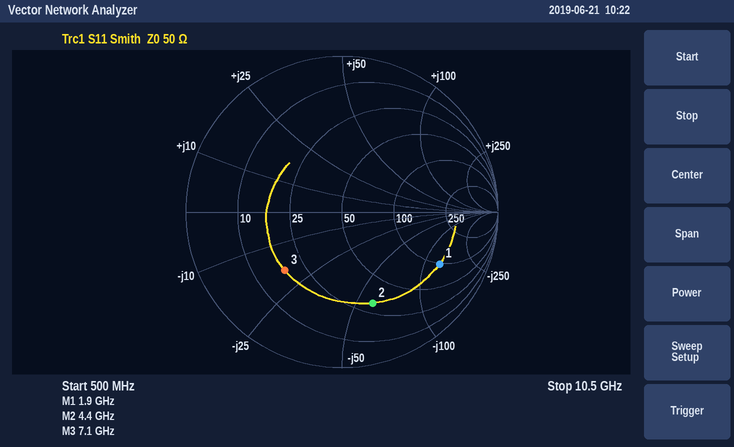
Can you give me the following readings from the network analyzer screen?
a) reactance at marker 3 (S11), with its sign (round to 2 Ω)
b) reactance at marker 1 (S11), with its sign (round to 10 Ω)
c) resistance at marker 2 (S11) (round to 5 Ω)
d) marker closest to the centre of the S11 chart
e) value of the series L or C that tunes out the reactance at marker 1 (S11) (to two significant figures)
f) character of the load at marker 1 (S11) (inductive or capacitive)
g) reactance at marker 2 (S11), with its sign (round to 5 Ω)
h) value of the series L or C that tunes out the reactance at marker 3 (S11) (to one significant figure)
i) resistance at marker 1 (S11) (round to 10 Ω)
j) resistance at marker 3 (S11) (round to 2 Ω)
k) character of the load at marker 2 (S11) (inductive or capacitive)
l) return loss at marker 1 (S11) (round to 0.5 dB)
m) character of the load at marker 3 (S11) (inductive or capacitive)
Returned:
-18 Ω
-130 Ω
30 Ω
marker 3
11 nH
capacitive
-60 Ω
400 pH
100 Ω
18 Ω
capacitive
3.0 dB
capacitive
